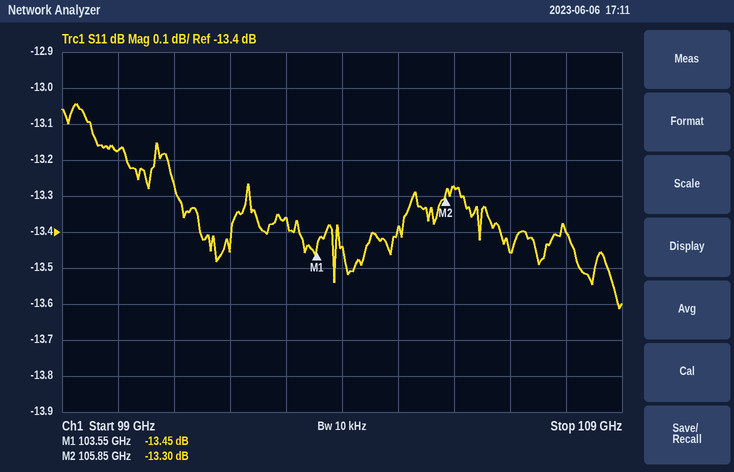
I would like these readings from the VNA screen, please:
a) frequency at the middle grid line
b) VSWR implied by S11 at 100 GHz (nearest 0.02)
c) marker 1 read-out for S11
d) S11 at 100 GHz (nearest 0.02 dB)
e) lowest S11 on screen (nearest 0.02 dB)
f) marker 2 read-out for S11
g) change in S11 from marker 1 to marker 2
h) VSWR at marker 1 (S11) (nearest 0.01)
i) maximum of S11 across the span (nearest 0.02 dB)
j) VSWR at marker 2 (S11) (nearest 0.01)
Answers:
104 GHz
1.56
-13.45 dB
-13.18 dB
-13.62 dB
-13.30 dB
0.15 dB
1.54
-13.04 dB
1.55
